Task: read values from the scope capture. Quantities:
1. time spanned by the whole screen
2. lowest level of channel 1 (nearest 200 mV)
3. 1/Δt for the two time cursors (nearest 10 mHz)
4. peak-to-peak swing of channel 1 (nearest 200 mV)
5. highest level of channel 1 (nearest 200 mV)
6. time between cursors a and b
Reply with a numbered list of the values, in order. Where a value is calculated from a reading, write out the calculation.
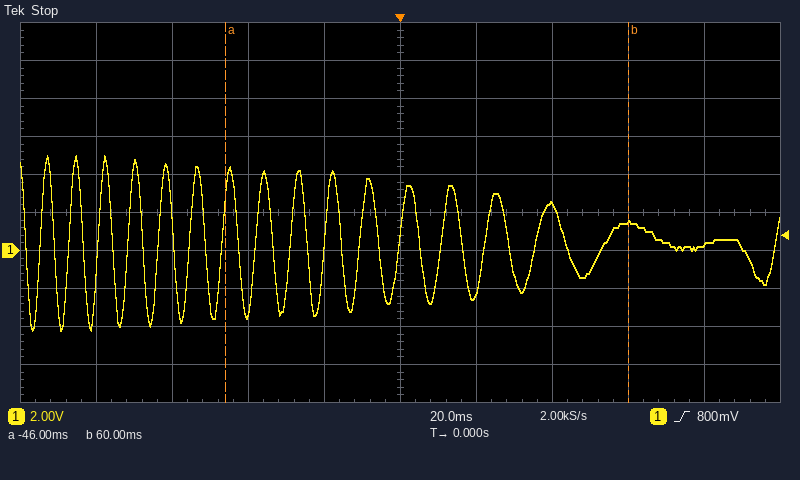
1. 200 ms
2. -4.2 V
3. 1 / 106 ms ≈ 9.43 Hz
4. 5.0 V − (-4.2 V) = 9.2 V
5. 5.0 V
6. 60 ms − (-46 ms) = 106 ms
